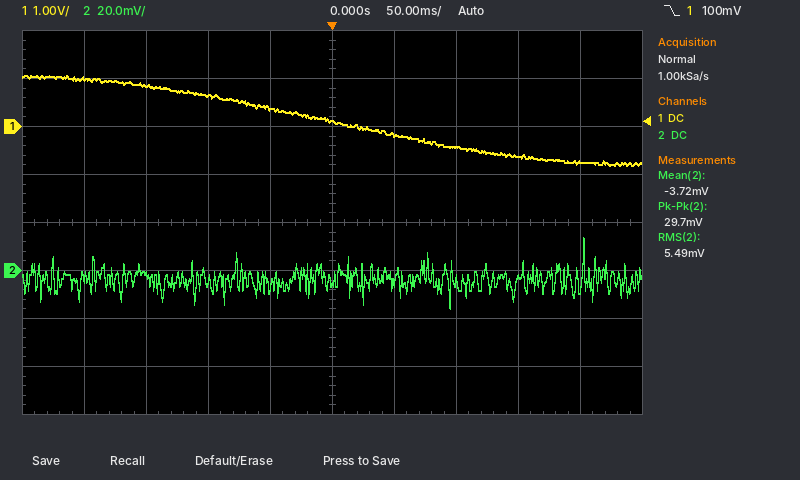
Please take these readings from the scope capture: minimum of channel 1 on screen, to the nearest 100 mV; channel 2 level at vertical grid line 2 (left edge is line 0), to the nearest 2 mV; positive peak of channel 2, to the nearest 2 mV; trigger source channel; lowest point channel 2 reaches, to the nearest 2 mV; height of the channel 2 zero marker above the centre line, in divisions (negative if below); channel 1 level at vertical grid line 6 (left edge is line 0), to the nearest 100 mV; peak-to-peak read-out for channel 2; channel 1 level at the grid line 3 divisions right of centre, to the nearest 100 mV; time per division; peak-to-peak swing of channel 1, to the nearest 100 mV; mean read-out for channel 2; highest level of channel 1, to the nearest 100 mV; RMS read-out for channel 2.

-800 mV
-2 mV
14 mV
channel 1
-16 mV
-1.0 div
-200 mV
29.7 mV
-600 mV
50 ms
1.9 V
-3.72 mV
1.1 V
5.49 mV
